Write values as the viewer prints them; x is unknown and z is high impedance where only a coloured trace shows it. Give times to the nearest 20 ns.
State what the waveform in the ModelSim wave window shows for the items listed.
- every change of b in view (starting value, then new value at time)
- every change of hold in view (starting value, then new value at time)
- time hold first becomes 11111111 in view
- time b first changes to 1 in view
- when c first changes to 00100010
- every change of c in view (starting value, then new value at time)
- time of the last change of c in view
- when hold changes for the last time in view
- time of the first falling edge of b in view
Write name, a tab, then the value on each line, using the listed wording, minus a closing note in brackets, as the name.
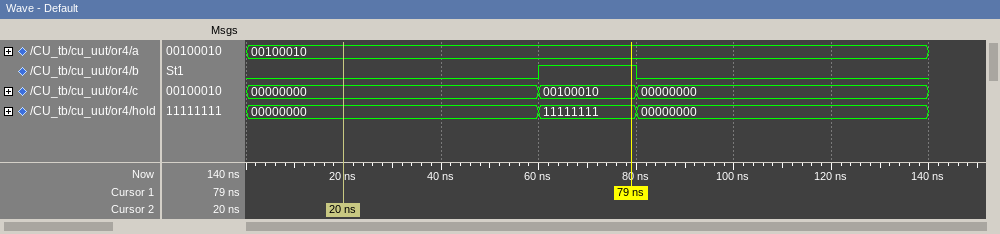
every change of b in view	0, 1 at 60 ns, 0 at 80 ns
every change of hold in view	00000000, 11111111 at 60 ns, 00000000 at 80 ns
time hold first becomes 11111111 in view	60 ns
time b first changes to 1 in view	60 ns
when c first changes to 00100010	60 ns
every change of c in view	00000000, 00100010 at 60 ns, 00000000 at 80 ns
time of the last change of c in view	80 ns
when hold changes for the last time in view	80 ns
time of the first falling edge of b in view	80 ns
